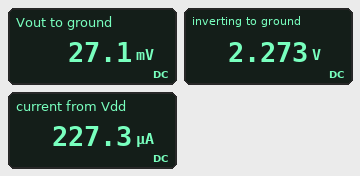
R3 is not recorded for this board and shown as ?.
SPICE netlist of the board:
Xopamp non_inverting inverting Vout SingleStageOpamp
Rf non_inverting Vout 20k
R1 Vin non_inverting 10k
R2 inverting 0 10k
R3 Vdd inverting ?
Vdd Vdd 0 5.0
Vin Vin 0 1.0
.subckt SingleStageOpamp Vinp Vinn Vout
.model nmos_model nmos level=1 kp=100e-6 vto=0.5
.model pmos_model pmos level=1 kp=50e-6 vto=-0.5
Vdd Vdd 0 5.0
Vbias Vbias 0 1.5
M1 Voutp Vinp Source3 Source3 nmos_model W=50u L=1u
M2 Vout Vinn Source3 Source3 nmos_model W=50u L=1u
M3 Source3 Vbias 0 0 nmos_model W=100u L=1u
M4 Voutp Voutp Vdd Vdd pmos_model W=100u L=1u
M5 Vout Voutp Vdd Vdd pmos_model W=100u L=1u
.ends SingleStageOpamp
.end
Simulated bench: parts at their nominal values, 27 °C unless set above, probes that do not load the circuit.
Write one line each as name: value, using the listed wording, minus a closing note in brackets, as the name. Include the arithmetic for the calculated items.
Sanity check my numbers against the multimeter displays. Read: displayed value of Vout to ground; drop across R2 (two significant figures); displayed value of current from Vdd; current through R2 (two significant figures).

displayed value of Vout to ground: 27.1 mV
drop across R2: 2.273 V = 2.3 V
displayed value of current from Vdd: 227.3 µA
current through R2: (2.273 V) / 10 kΩ = 230 µA
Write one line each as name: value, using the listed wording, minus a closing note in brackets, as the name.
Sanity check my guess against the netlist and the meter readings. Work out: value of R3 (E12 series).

value of R3: 12 kΩ
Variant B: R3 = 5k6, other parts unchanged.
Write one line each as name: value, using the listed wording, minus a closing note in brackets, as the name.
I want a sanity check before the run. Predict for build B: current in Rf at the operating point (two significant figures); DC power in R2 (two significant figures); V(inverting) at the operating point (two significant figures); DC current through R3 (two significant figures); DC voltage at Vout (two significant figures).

current in Rf at the operating point: 33 µA
DC power in R2: 1.0 mW
V(inverting) at the operating point: 3.2 V
DC current through R3: 320 µA
DC voltage at Vout: 23 mV
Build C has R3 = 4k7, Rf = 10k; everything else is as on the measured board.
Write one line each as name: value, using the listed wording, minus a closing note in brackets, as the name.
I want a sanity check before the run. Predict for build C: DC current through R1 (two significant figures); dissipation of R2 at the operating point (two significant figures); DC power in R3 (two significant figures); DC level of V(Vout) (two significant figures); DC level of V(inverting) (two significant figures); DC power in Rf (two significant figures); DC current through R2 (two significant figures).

DC current through R1: 50 µA
dissipation of R2 at the operating point: 1.2 mW
DC power in R3: 540 µW
DC level of V(Vout): 8.4 mV
DC level of V(inverting): 3.4 V
DC power in Rf: 25 µW
DC current through R2: 340 µA
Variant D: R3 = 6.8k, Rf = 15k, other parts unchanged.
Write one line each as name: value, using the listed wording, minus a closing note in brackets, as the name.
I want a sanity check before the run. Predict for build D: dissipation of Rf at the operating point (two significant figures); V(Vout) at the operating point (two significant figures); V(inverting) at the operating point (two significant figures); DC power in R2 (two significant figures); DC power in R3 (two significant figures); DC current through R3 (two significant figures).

dissipation of Rf at the operating point: 23 µW
V(Vout) at the operating point: 14 mV
V(inverting) at the operating point: 3.0 V
DC power in R2: 890 µW
DC power in R3: 600 µW
DC current through R3: 300 µA
